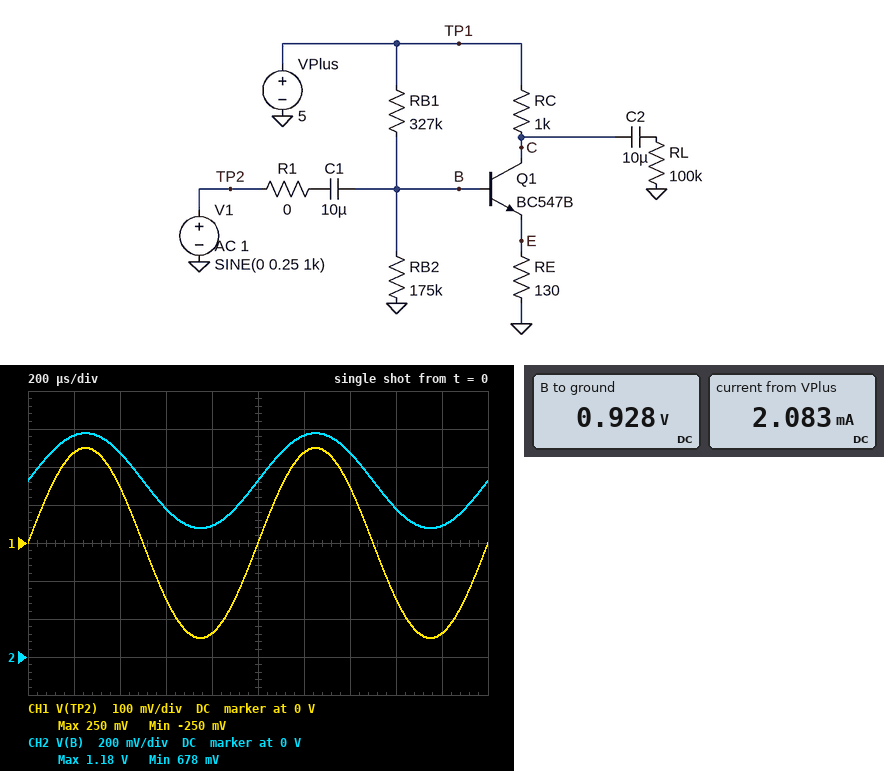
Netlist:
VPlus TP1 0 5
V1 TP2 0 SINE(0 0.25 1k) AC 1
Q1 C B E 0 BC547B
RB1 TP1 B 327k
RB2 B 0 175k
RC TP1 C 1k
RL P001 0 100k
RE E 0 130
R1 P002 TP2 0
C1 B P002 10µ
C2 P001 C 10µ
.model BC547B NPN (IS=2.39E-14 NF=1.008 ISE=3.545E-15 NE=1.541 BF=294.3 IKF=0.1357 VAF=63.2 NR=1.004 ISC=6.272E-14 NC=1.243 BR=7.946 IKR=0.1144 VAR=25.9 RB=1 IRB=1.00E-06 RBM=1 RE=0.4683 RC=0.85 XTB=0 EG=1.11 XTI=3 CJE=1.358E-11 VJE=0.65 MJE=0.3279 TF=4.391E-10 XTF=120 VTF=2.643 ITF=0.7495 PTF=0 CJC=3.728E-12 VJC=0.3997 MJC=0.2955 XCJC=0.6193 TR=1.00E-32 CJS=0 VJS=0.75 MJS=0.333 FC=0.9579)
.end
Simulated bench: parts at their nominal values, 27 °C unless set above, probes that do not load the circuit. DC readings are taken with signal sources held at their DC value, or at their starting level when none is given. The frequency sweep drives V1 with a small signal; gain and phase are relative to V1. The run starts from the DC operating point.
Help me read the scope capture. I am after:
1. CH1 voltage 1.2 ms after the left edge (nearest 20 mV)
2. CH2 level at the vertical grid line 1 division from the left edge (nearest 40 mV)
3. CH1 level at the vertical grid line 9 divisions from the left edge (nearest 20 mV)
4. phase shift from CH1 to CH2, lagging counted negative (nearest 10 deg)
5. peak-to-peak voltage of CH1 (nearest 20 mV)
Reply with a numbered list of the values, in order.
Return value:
1. 240 mV
2. 1.16 V
3. -240 mV
4. 0 deg
5. 500 mV
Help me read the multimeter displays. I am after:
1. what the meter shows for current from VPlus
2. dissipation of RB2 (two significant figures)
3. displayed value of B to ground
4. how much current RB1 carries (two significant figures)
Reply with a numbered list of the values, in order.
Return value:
1. 2.083 mA
2. 4.9 µW
3. 0.928 V
4. 12 µA
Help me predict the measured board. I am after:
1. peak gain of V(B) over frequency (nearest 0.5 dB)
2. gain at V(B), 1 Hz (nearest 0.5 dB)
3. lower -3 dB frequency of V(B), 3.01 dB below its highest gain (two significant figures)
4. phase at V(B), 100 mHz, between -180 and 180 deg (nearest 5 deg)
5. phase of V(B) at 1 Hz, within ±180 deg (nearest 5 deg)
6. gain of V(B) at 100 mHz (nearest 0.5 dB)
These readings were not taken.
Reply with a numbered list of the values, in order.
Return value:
1. 0 dB
2. -1.0 dB
3. 540 mHz
4. 80 deg
5. 30 deg
6. -15.0 dB
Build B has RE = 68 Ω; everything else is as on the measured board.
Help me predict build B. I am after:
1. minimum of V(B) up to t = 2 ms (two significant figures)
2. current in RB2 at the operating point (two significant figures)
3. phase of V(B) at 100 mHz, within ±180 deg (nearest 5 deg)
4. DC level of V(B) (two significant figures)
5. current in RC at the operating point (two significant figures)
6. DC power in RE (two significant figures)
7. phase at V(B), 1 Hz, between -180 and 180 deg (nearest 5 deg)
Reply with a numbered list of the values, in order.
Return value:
1. 550 mV
2. 4.7 µA
3. 85 deg
4. 820 mV
5. 2.3 mA
6. 370 µW
7. 40 deg
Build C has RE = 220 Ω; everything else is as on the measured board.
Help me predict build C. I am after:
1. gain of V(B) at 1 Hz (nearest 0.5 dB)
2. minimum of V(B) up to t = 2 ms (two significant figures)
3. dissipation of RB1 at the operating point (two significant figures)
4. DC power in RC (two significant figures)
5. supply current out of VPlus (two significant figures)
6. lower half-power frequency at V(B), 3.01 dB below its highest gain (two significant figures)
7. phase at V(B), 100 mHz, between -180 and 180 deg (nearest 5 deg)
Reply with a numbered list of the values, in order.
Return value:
1. -0.5 dB
2. 800 mV
3. 48 µW
4. 3.2 mW
5. 1.8 mA
6. 380 mHz
7. 75 deg
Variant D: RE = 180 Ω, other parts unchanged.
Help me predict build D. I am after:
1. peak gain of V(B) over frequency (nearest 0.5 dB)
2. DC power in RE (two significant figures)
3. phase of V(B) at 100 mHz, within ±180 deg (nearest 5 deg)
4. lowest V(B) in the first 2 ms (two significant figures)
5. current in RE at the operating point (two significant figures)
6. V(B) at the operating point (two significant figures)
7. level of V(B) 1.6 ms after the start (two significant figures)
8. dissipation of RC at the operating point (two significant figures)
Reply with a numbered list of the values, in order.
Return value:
1. 0 dB
2. 650 µW
3. 75 deg
4. 750 mV
5. 1.9 mA
6. 1.0 V
7. 850 mV
8. 3.6 mW
